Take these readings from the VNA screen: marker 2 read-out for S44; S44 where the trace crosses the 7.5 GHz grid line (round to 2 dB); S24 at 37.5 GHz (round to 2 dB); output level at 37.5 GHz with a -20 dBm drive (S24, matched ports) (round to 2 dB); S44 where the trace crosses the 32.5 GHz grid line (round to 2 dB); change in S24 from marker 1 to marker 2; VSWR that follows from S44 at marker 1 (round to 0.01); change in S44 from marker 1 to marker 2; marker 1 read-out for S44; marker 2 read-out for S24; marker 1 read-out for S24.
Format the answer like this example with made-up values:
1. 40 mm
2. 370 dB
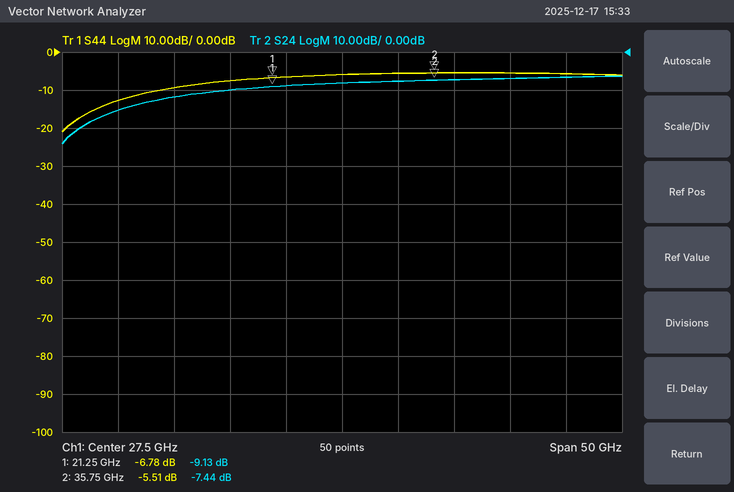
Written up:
1. -5.51 dB
2. -12 dB
3. -8 dB
4. -28 dBm
5. -6 dB
6. 1.69 dB
7. 2.69
8. 1.27 dB
9. -6.78 dB
10. -7.44 dB
11. -9.13 dB
